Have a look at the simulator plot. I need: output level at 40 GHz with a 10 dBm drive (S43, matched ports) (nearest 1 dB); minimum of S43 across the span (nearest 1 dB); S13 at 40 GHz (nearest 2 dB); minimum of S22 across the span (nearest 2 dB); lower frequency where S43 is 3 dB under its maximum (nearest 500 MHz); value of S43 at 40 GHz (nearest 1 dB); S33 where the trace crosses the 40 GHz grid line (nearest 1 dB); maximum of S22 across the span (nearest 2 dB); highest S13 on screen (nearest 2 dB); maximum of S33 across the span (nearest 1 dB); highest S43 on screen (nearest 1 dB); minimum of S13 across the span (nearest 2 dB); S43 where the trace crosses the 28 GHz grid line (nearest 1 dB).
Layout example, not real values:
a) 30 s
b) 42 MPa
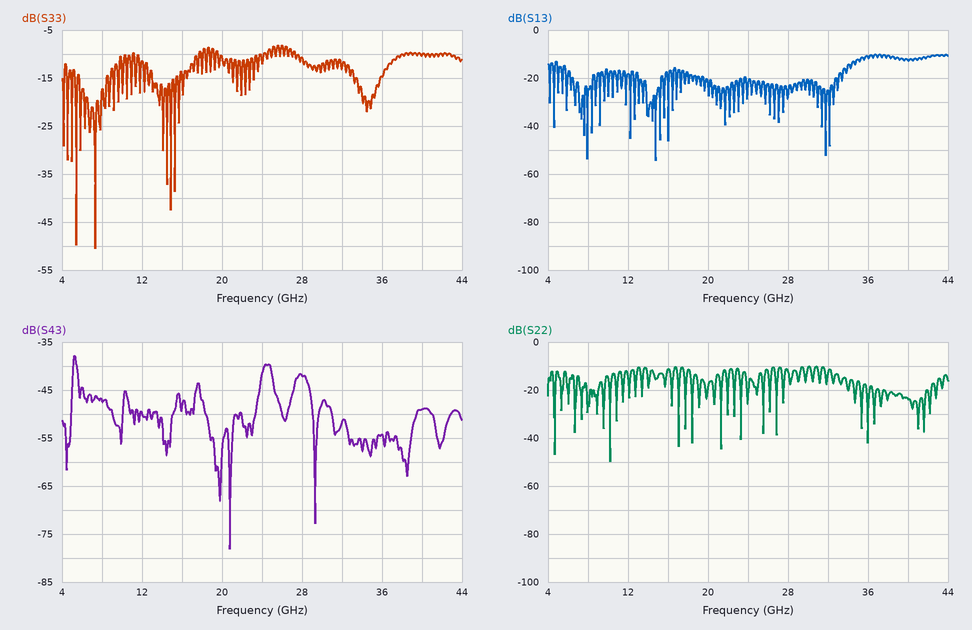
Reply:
a) -39 dBm
b) -78 dB
c) -12 dB
d) -50 dB
e) 5.0 GHz
f) -49 dB
g) -10 dB
h) -10 dB
i) -10 dB
j) -8 dB
k) -38 dB
l) -54 dB
m) -42 dB
